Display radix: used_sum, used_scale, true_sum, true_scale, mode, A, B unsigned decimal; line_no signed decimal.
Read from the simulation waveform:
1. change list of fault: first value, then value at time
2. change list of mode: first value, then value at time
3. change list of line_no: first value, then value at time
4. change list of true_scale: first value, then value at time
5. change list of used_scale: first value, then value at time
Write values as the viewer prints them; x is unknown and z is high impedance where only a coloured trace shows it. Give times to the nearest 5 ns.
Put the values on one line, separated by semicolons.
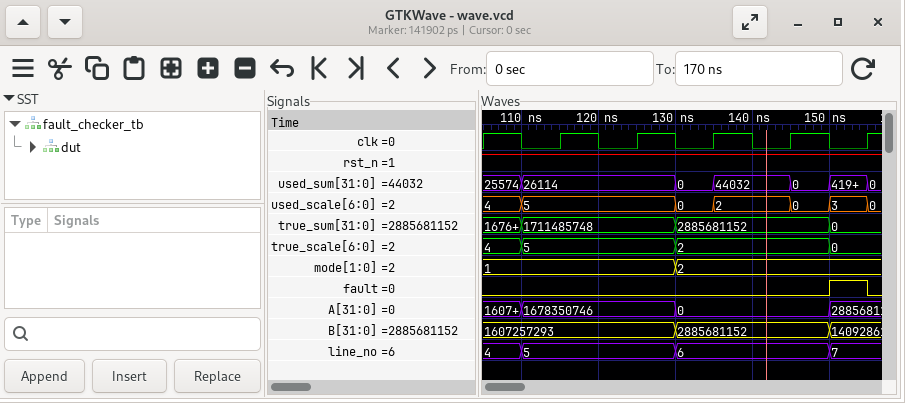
0, 1 at 150 ns, 0 at 155 ns; 1, 2 at 130 ns; 4, 5 at 110 ns, 6 at 130 ns, 7 at 150 ns; 4, 5 at 110 ns, 2 at 130 ns, 0 at 150 ns; 4, 5 at 110 ns, 0 at 130 ns, 2 at 135 ns, 0 at 145 ns, 3 at 150 ns, 0 at 155 ns
